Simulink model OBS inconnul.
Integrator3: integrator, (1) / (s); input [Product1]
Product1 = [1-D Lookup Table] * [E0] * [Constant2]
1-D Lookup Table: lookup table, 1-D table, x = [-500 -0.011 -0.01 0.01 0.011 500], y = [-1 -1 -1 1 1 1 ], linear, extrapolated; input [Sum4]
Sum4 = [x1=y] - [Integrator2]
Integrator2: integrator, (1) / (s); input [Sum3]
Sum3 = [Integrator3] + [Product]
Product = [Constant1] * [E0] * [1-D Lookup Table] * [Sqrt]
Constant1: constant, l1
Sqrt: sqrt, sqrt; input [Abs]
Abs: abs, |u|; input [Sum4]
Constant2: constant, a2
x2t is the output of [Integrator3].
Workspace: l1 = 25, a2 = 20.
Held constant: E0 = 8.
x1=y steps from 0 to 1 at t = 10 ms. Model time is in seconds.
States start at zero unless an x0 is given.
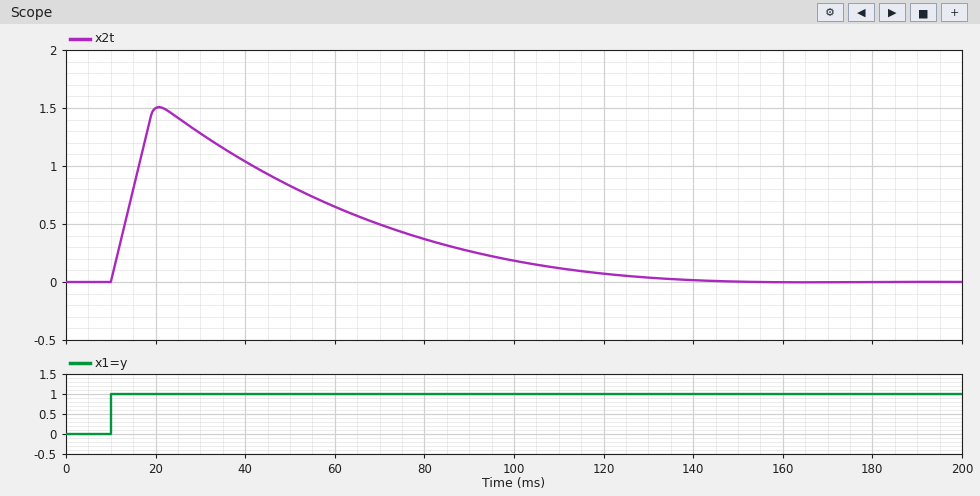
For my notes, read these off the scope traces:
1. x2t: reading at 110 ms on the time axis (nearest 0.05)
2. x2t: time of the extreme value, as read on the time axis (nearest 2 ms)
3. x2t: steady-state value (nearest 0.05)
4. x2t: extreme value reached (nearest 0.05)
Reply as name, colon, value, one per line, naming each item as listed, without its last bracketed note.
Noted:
x2t: reading at 110 ms on the time axis: 0.10
x2t: time of the extreme value, as read on the time axis: 20 ms
x2t: steady-state value: 0.00
x2t: extreme value reached: 1.50
